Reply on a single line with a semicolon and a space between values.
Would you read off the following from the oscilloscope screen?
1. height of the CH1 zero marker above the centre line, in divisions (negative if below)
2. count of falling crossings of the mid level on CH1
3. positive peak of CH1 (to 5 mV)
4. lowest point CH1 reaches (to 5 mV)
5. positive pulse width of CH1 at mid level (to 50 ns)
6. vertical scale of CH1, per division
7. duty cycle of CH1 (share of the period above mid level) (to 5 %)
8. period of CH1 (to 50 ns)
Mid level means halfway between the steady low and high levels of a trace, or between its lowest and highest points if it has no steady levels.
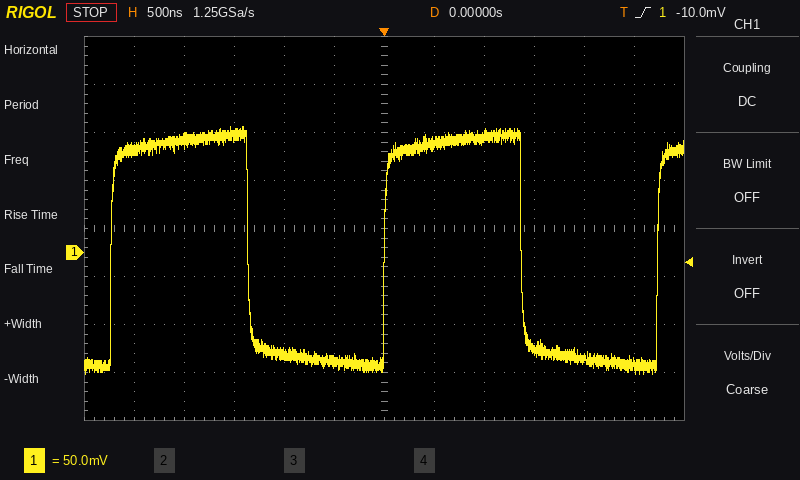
-0.5 div; 2; 130 mV; -125 mV; 1.35 µs; 50 mV; 50 %; 2.75 µs
